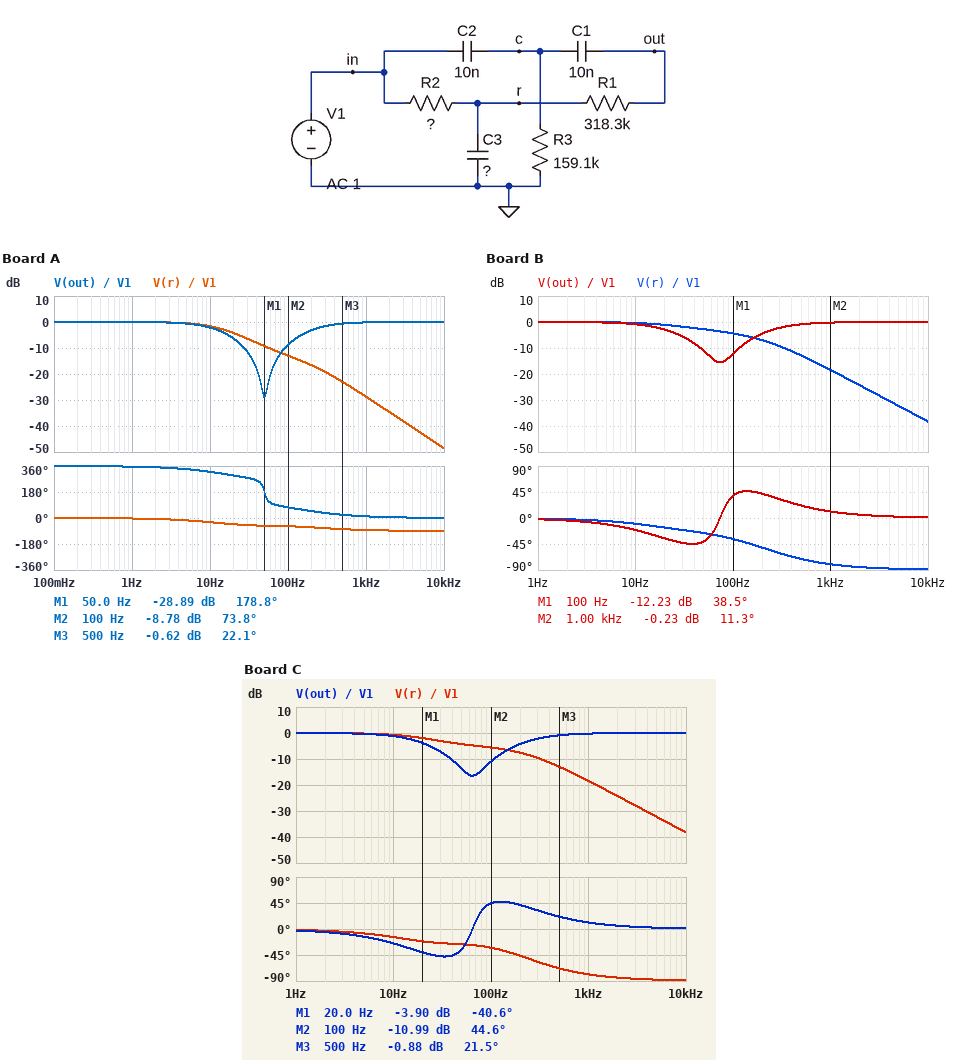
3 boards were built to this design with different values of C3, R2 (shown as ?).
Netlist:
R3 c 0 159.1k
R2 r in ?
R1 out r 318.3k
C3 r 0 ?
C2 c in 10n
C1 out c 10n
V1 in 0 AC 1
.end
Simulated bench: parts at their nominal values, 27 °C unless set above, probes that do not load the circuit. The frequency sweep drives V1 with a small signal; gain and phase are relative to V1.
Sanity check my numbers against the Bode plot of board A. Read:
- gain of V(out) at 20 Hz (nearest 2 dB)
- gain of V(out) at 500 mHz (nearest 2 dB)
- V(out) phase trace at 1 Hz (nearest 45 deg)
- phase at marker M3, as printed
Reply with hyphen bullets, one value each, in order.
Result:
- -6 dB
- 0 dB
- 360 deg
- 22.1 deg
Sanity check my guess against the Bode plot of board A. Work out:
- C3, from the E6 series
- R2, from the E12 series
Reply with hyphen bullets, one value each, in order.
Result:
- 33 nF
- 220 kΩ
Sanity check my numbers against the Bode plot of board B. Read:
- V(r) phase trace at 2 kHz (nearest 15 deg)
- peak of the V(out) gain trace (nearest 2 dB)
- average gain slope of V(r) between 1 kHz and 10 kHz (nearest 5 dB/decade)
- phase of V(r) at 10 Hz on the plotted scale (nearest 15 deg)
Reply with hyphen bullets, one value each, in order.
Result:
- -90 deg
- 0 dB
- -20 dB/decade
- -15 deg
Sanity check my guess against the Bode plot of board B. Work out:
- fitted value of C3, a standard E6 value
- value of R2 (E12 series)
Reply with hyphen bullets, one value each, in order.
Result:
- 15 nF
- 120 kΩ
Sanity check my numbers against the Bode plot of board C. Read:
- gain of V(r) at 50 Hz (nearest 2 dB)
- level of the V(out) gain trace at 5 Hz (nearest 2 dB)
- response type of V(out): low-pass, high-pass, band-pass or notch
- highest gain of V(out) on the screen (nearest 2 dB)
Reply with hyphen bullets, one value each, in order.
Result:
- -4 dB
- 0 dB
- notch
- 0 dB
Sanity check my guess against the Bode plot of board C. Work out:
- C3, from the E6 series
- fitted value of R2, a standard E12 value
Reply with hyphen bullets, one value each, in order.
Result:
- 10 nF
- 220 kΩ
